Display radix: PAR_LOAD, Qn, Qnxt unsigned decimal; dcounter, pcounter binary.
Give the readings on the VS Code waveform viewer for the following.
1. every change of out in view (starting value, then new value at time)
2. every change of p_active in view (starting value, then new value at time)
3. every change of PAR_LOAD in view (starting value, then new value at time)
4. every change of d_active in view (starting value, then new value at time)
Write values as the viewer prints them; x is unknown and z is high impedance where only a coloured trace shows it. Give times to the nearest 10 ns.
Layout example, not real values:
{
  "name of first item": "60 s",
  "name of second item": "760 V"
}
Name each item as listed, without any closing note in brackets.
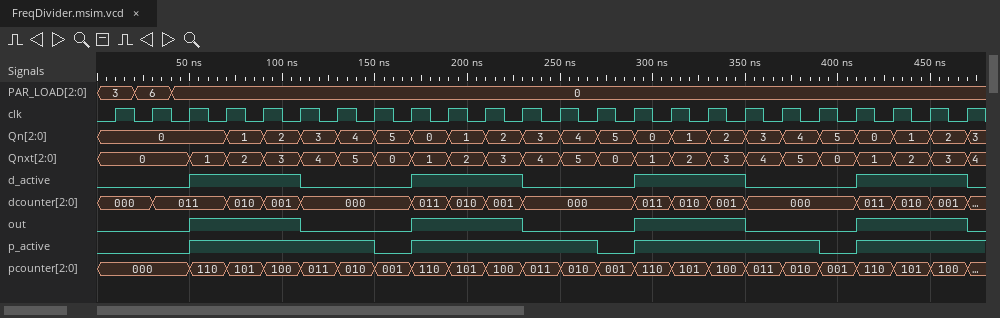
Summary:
{
  "every change of out in view": "0, 1 at 50 ns, 0 at 110 ns, 1 at 170 ns, 0 at 230 ns, 1 at 290 ns, 0 at 350 ns, 1 at 410 ns, 0 at 470 ns",
  "every change of p_active in view": "0, 1 at 50 ns, 0 at 150 ns, 1 at 170 ns, 0 at 270 ns, 1 at 290 ns, 0 at 390 ns, 1 at 410 ns",
  "every change of PAR_LOAD in view": "3, 6 at 20 ns, 0 at 40 ns",
  "every change of d_active in view": "0, 1 at 50 ns, 0 at 110 ns, 1 at 170 ns, 0 at 230 ns, 1 at 290 ns, 0 at 350 ns, 1 at 410 ns, 0 at 470 ns"
}
